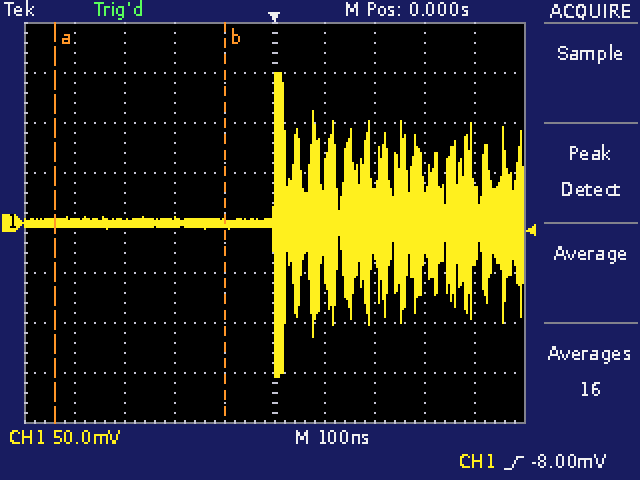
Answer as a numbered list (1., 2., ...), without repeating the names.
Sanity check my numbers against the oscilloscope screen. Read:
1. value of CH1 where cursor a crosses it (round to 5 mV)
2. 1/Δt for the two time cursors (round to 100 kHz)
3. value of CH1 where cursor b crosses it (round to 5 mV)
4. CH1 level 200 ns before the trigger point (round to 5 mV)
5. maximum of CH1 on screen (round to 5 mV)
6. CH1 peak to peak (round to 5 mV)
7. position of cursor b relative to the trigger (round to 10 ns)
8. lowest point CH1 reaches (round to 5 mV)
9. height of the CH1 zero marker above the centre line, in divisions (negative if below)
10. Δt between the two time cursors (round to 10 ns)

1. 0 mV
2. 2.9 MHz
3. 0 mV
4. 0 mV
5. 150 mV
6. 305 mV
7. -100 ns
8. -155 mV
9. 0.0 div
10. 340 ns
